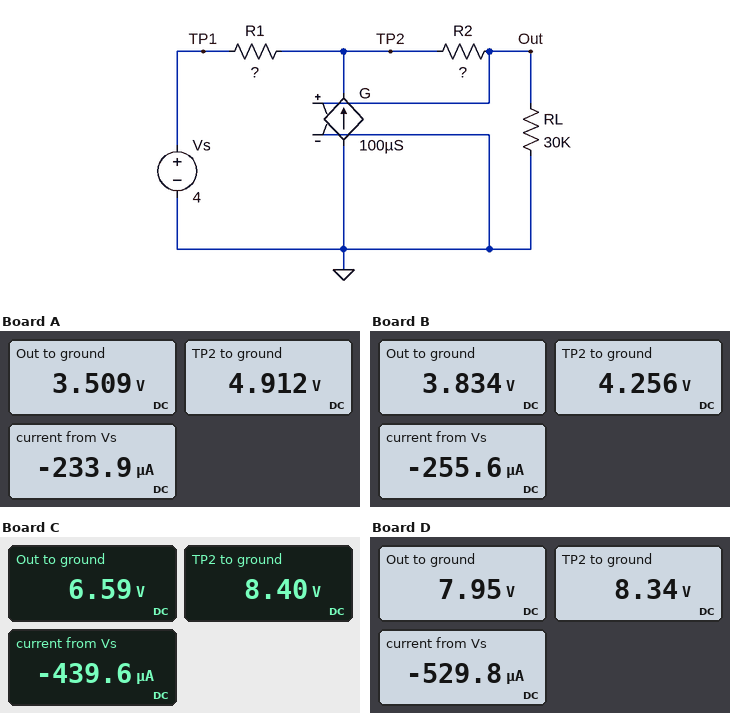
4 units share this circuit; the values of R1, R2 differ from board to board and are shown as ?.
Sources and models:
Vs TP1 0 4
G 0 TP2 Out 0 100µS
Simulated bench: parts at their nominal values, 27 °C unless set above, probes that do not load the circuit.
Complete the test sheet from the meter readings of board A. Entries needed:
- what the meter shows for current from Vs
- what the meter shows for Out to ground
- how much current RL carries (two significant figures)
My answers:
-233.9 µA
3.509 V
120 µA
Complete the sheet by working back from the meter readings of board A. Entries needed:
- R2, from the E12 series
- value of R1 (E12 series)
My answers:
12 kΩ
3.9 kΩ
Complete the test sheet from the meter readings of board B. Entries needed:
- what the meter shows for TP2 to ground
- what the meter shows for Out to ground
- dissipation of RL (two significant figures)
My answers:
4.256 V
3.834 V
490 µW
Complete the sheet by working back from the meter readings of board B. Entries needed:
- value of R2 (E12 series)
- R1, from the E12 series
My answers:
3.3 kΩ
1 kΩ
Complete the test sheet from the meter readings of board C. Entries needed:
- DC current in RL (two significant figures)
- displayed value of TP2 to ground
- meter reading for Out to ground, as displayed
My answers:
220 µA
8.40 V
6.59 V
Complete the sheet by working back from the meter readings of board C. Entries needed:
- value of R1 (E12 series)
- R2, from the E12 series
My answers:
10 kΩ
8.2 kΩ
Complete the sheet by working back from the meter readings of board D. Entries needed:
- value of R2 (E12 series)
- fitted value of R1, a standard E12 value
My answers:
1.5 kΩ
8.2 kΩ
